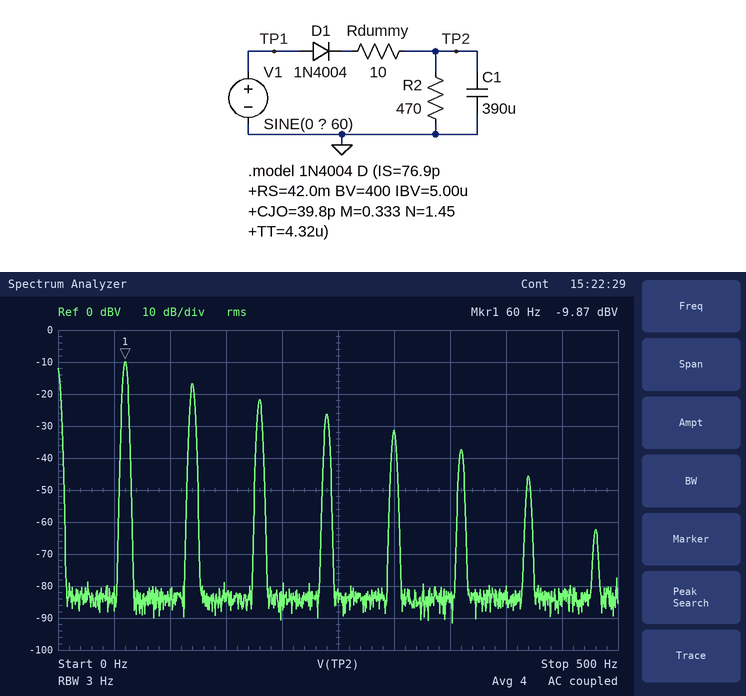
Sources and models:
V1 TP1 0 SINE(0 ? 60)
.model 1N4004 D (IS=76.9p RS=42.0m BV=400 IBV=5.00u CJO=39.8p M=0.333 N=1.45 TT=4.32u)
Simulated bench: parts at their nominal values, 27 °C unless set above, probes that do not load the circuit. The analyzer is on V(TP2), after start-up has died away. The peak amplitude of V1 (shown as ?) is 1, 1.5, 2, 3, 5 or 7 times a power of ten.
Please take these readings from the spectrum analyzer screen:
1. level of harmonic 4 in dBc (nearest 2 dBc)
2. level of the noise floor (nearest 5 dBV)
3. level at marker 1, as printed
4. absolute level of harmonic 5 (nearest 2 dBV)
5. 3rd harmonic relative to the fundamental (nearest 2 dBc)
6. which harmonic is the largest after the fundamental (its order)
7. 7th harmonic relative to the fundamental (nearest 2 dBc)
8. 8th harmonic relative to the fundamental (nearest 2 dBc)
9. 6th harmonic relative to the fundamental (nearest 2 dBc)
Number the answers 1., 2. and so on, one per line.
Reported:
1. -16 dBc
2. -85 dBV
3. -9.87 dBV
4. -32 dBV
5. -12 dBc
6. 2
7. -36 dBc
8. -52 dBc
9. -28 dBc
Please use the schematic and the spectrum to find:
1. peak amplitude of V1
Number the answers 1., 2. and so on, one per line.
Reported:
1. 20 V
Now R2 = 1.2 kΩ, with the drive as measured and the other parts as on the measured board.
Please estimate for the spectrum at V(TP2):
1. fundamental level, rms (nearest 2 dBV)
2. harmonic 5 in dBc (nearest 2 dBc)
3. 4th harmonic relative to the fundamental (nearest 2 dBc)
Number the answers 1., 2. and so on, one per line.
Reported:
1. -18 dBV
2. -18 dBc
3. -14 dBc
